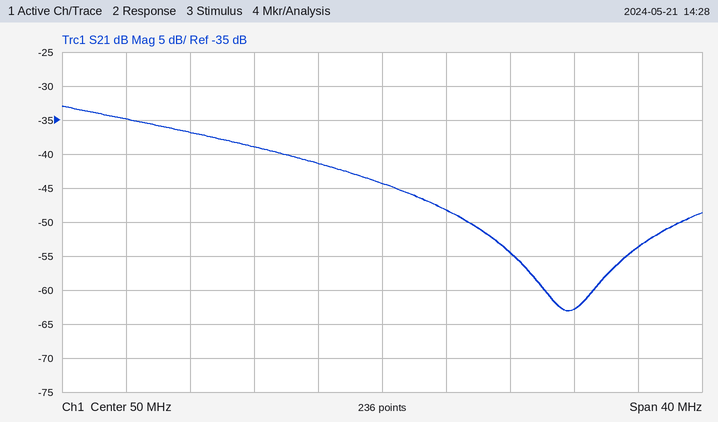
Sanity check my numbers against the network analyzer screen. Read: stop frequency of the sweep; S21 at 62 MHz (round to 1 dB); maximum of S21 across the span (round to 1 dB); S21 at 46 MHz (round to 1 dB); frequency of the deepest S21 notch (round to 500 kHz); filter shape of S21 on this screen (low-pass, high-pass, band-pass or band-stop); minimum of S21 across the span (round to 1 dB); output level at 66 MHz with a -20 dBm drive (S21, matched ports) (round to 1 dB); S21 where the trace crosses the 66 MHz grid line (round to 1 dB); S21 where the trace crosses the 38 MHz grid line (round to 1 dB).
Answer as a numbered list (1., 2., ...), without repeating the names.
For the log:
1. 70 MHz
2. -63 dB
3. -33 dB
4. -41 dB
5. 61.5 MHz
6. low-pass
7. -63 dB
8. -74 dBm
9. -54 dB
10. -37 dB
